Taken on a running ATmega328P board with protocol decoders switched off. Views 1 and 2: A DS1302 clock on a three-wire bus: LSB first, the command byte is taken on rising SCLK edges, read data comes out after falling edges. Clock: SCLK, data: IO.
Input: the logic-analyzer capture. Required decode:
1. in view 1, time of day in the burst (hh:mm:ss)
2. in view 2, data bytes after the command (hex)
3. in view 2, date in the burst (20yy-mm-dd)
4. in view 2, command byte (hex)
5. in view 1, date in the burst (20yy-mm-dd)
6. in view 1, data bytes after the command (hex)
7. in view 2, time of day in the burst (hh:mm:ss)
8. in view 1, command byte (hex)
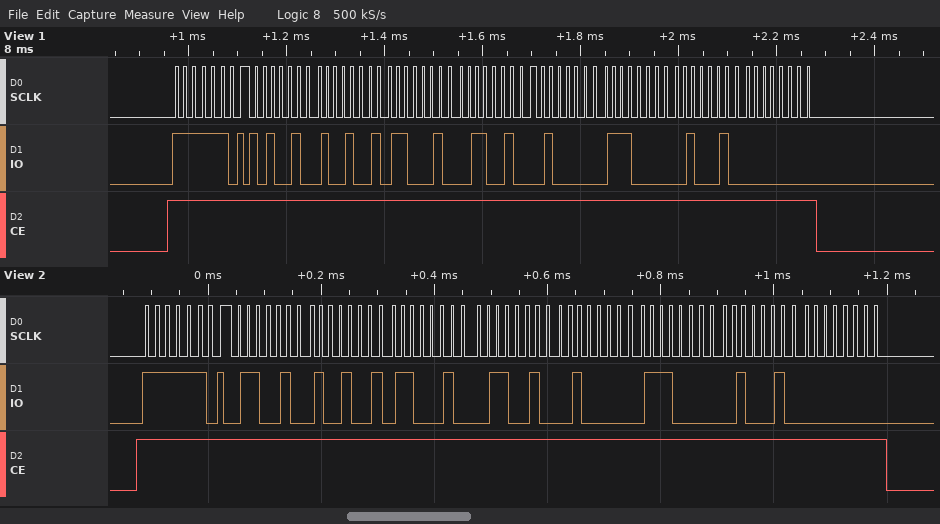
23:49:25
26 49 23 26 02 07 22 00
2022-02-26
0xBF
2022-02-26
25 49 23 26 02 07 22 00
23:49:26
0xBF
